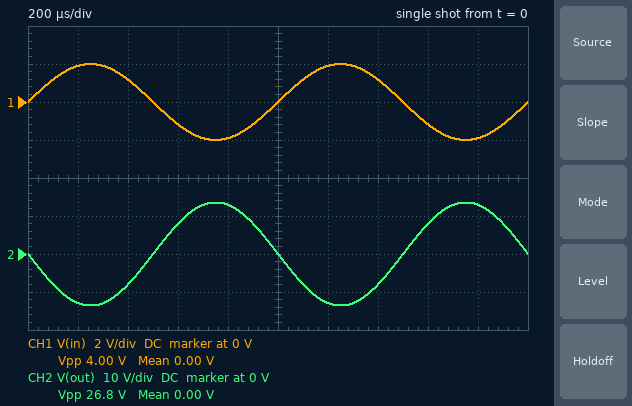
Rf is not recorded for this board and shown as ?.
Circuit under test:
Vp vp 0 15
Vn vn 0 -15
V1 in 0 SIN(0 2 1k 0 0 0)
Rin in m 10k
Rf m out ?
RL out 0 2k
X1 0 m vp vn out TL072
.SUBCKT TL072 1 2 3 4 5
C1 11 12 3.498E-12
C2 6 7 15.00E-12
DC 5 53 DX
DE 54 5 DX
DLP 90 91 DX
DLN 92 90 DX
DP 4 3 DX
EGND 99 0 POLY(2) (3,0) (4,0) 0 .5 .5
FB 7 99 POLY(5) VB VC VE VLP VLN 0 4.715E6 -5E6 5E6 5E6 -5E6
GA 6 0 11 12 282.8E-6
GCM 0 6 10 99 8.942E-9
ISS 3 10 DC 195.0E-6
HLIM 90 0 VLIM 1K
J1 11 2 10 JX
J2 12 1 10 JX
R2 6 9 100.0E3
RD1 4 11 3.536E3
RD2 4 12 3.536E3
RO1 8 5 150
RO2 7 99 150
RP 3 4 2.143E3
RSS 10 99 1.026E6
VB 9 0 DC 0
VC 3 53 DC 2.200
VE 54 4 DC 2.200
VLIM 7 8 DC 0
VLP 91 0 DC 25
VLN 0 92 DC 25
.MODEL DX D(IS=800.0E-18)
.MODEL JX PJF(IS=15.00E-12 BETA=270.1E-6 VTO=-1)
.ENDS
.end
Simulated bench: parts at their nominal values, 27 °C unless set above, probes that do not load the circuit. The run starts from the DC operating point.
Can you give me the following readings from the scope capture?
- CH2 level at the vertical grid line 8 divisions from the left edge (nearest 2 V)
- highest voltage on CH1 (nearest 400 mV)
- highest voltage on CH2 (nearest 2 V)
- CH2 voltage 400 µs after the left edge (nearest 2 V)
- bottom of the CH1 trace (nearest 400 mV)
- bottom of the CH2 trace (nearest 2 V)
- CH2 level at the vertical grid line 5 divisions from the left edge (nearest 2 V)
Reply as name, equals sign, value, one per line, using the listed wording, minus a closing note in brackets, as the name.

CH2 level at the vertical grid line 8 divisions from the left edge = 8 V
highest voltage on CH1 = 2.0 V
highest voltage on CH2 = 14 V
CH2 voltage 400 µs after the left edge = -8 V
bottom of the CH1 trace = -2.0 V
bottom of the CH2 trace = -14 V
CH2 level at the vertical grid line 5 divisions from the left edge = 0 V
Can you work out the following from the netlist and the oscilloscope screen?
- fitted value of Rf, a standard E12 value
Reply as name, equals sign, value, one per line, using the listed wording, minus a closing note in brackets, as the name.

fitted value of Rf, a standard E12 value = 68 kΩ
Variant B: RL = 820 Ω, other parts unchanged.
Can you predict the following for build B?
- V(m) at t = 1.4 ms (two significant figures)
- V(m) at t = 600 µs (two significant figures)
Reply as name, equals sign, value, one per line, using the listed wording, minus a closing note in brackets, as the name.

V(m) at t = 1.4 ms = -3.7 mV
V(m) at t = 600 µs = -3.8 mV
